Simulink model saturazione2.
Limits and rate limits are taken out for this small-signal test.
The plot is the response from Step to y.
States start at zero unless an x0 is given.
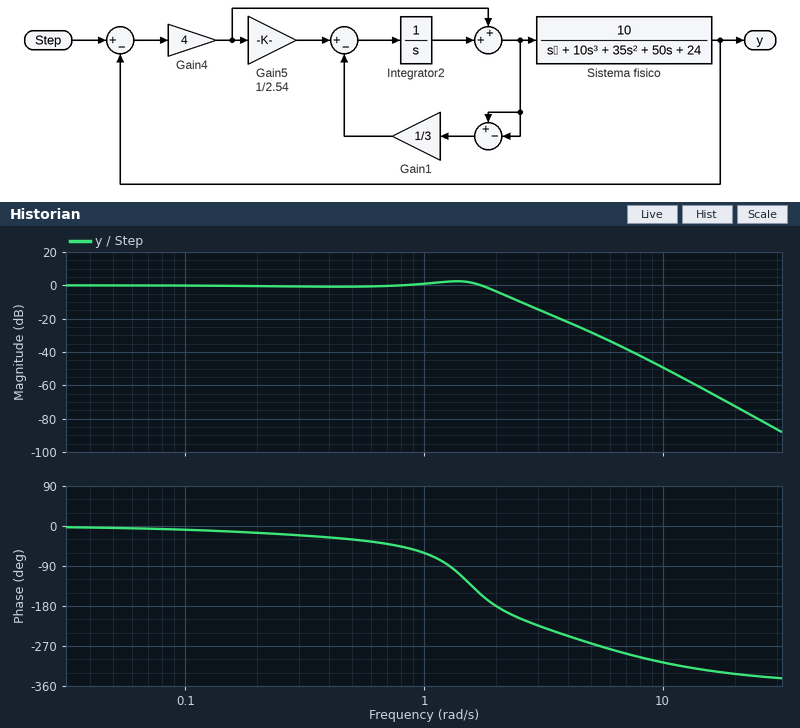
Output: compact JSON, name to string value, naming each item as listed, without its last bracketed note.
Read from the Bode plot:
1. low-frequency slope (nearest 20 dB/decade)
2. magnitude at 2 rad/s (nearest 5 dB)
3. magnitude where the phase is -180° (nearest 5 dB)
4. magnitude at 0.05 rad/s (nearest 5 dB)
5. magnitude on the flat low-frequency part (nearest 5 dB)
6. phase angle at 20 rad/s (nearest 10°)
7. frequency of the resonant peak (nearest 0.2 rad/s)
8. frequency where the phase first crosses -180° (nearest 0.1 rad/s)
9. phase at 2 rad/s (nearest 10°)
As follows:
{"low-frequency slope": "0 dB/decade", "magnitude at 2 rad/s": "-5 dB", "magnitude where the phase is -180°": "-5 dB", "magnitude at 0.05 rad/s": "0 dB", "magnitude on the flat low-frequency part": "0 dB", "phase angle at 20 rad/s": "-330°", "frequency of the resonant peak": "1.4 rad/s", "frequency where the phase first crosses -180°": "2.0 rad/s", "phase at 2 rad/s": "-180°"}
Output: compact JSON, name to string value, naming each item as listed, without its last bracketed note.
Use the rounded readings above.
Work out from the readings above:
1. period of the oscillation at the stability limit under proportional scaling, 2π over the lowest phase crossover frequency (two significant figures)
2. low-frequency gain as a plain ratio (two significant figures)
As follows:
{"period of the oscillation at the stability limit under proportional scaling, 2π over the lowest phase crossover frequency": "3.1 s", "low-frequency gain as a plain ratio": "1.0"}
